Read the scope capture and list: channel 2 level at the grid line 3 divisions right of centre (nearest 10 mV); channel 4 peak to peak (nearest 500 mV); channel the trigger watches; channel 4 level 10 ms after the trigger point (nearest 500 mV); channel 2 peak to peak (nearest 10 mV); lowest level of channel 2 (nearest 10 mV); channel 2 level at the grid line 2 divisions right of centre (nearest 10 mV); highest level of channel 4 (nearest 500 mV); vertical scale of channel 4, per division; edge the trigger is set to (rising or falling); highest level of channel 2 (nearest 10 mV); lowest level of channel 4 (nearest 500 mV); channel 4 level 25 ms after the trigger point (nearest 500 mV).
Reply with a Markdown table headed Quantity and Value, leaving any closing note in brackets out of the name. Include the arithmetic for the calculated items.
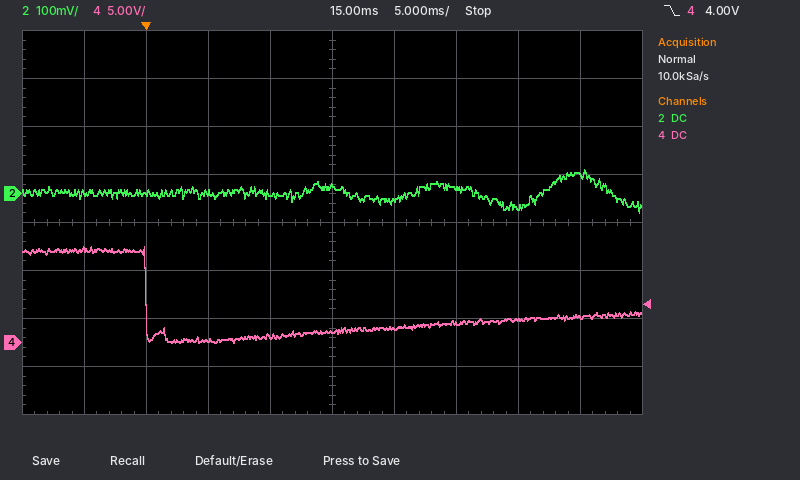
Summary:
| Quantity | Value |
|---|---|
| channel 2 level at the grid line 3 divisions right of centre | -30 mV |
| channel 4 peak to peak | 10.0 V − (0.0 V) = 10.0 V |
| channel the trigger watches | channel 4 |
| channel 4 level 10 ms after the trigger point | 500 mV |
| channel 2 peak to peak | 50 mV − (-40 mV) = 90 mV |
| lowest level of channel 2 | -40 mV |
| channel 2 level at the grid line 2 divisions right of centre | 10 mV |
| highest level of channel 4 | 10.0 V |
| vertical scale of channel 4, per division | 5 V |
| edge the trigger is set to | falling |
| highest level of channel 2 | 50 mV |
| lowest level of channel 4 | 0.0 V |
| channel 4 level 25 ms after the trigger point | 2.0 V |
